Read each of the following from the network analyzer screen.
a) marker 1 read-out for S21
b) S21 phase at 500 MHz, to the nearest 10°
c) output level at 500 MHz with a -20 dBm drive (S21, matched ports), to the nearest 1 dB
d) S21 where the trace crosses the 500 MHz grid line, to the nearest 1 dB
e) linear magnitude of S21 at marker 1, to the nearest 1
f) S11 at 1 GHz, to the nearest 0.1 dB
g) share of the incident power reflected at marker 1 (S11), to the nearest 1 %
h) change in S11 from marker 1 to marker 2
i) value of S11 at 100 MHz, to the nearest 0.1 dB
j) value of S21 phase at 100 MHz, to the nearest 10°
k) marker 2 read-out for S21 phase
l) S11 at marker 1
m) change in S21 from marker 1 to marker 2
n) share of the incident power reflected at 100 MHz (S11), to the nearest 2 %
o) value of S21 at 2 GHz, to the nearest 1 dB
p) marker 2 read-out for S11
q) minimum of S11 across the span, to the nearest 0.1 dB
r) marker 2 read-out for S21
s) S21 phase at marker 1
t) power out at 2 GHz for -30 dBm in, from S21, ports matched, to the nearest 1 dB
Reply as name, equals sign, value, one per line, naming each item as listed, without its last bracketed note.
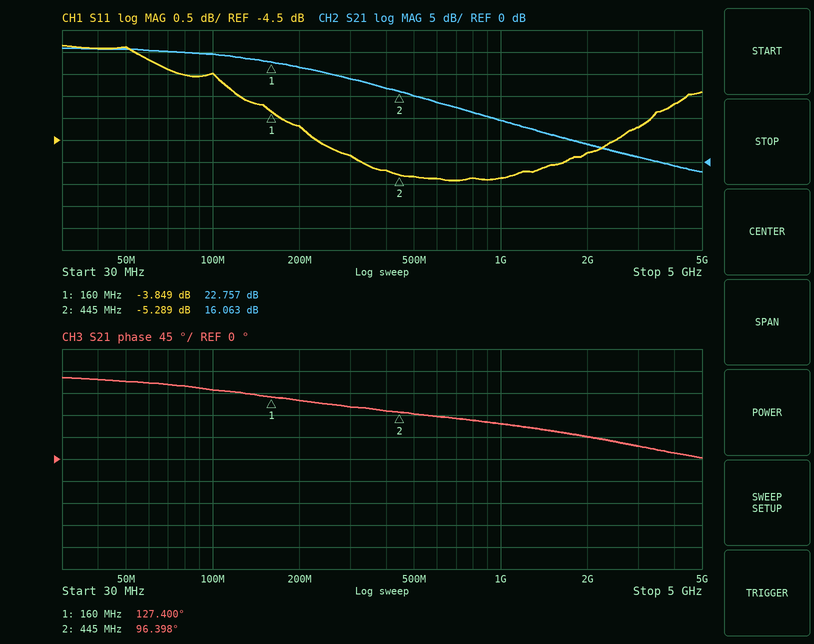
marker 1 read-out for S21 = 22.757 dB
S21 phase at 500 MHz, to the nearest 10° = 90°
output level at 500 MHz with a -20 dBm drive (S21, matched ports), to the nearest 1 dB = -5 dBm
S21 where the trace crosses the 500 MHz grid line, to the nearest 1 dB = 15 dB
linear magnitude of S21 at marker 1, to the nearest 1 = 14
S11 at 1 GHz, to the nearest 0.1 dB = -5.4 dB
share of the incident power reflected at marker 1 (S11), to the nearest 1 % = 41 %
change in S11 from marker 1 to marker 2 = -1.440 dB
value of S11 at 100 MHz, to the nearest 0.1 dB = -3.0 dB
value of S21 phase at 100 MHz, to the nearest 10° = 140°
marker 2 read-out for S21 phase = 96.398°
S11 at marker 1 = -3.849 dB
change in S21 from marker 1 to marker 2 = -6.694 dB
share of the incident power reflected at 100 MHz (S11), to the nearest 2 % = 50 %
value of S21 at 2 GHz, to the nearest 1 dB = 4 dB
marker 2 read-out for S11 = -5.289 dB
minimum of S11 across the span, to the nearest 0.1 dB = -5.4 dB
marker 2 read-out for S21 = 16.063 dB
S21 phase at marker 1 = 127.400°
power out at 2 GHz for -30 dBm in, from S21, ports matched, to the nearest 1 dB = -26 dBm
